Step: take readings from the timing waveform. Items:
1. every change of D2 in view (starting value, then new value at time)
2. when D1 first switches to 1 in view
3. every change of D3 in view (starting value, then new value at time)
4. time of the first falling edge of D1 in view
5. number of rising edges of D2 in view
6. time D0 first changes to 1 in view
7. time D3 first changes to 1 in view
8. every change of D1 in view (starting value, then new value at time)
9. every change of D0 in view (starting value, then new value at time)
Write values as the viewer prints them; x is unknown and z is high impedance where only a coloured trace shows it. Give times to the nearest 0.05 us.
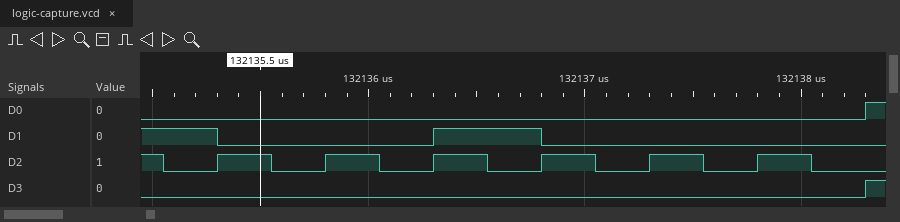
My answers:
1, 0 at 132135.05 us, 1 at 132135.3 us, 0 at 132135.55 us, 1 at 132135.8 us, 0 at 132136.05 us, 1 at 132136.3 us, 0 at 132136.55 us, 1 at 132136.8 us, 0 at 132137.05 us, 1 at 132137.3 us, 0 at 132137.55 us, 1 at 132137.8 us, 0 at 132138.05 us
132136.3 us
0, 1 at 132138.3 us
132135.3 us
6
132138.3 us
132138.3 us
1, 0 at 132135.3 us, 1 at 132136.3 us, 0 at 132136.8 us
0, 1 at 132138.3 us
